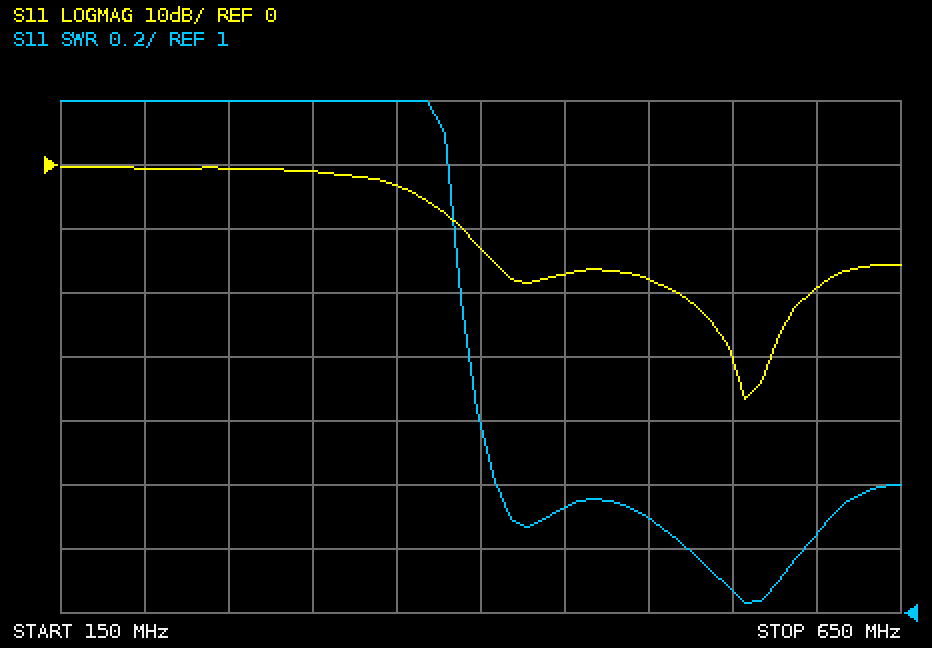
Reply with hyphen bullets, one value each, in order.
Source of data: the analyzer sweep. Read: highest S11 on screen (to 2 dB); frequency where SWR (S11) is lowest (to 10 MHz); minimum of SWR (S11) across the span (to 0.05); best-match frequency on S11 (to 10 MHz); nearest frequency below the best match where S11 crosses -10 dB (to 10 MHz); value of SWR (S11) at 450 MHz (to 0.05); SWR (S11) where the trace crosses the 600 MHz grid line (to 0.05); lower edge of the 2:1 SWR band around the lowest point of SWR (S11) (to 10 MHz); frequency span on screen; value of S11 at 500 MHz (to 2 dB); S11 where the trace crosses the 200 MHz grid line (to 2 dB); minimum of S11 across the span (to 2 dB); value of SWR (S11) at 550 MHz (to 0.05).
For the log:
- 0 dB
- 560 MHz
- 1.05
- 560 MHz
- 390 MHz
- 1.35
- 1.25
- 390 MHz
- 500 MHz
- -18 dB
- 0 dB
- -36 dB
- 1.05
